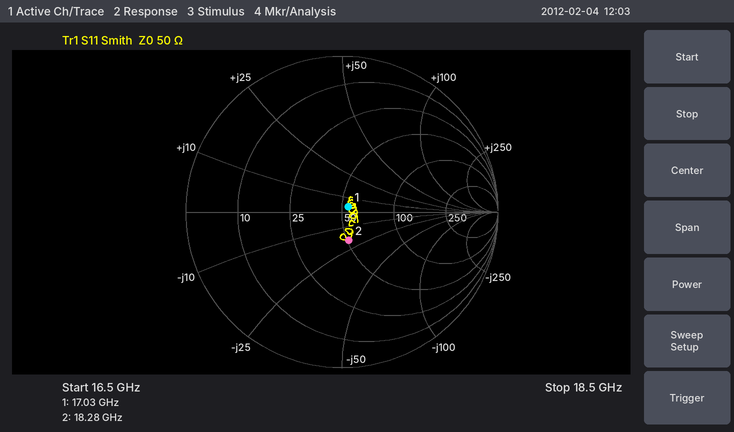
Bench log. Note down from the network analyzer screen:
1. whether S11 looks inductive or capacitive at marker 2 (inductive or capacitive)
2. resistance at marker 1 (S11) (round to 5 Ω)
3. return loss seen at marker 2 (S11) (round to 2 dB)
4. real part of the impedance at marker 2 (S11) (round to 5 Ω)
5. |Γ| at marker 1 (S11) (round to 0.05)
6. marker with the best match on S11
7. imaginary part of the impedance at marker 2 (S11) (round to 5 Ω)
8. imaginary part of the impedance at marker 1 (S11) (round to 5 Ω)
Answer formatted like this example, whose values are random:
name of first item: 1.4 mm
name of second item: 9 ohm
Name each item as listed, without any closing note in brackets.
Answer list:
whether S11 looks inductive or capacitive at marker 2: capacitive
resistance at marker 1 (S11): 55 Ω
return loss seen at marker 2 (S11): 14 dB
real part of the impedance at marker 2 (S11): 50 Ω
|Γ| at marker 1 (S11): 0.05
marker with the best match on S11: marker 1
imaginary part of the impedance at marker 2 (S11): -20 Ω
imaginary part of the impedance at marker 1 (S11): +5 Ω
